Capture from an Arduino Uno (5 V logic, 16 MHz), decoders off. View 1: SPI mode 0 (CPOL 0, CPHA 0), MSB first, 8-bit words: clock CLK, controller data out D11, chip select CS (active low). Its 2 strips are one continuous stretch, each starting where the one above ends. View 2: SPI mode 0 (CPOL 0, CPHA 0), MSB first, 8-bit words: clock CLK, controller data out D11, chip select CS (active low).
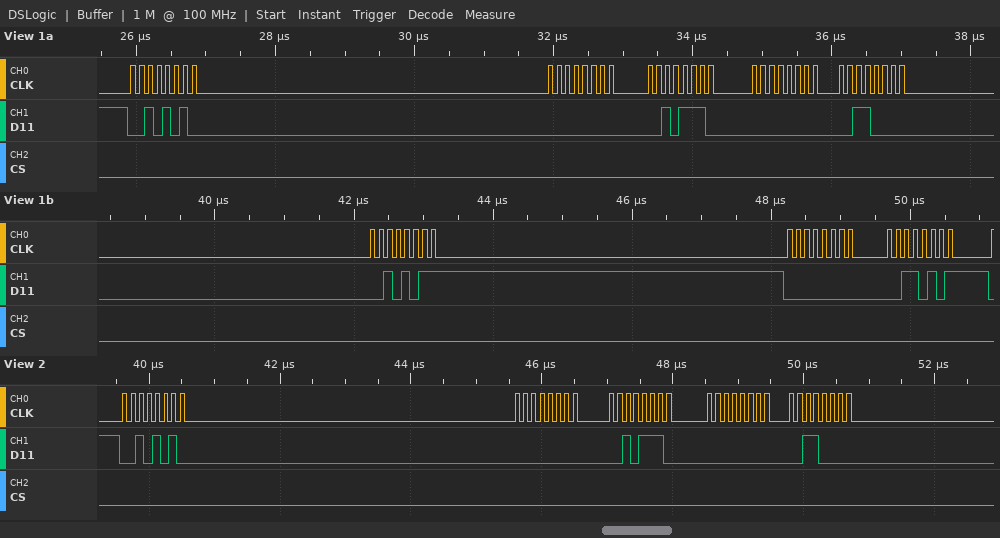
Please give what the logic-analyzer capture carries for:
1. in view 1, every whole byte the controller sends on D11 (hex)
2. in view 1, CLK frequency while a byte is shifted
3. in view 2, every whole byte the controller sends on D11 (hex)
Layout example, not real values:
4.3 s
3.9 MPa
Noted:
2A 00 2E 00 30 2B 00 35
8 MHz
2A 00 2E 00 30
